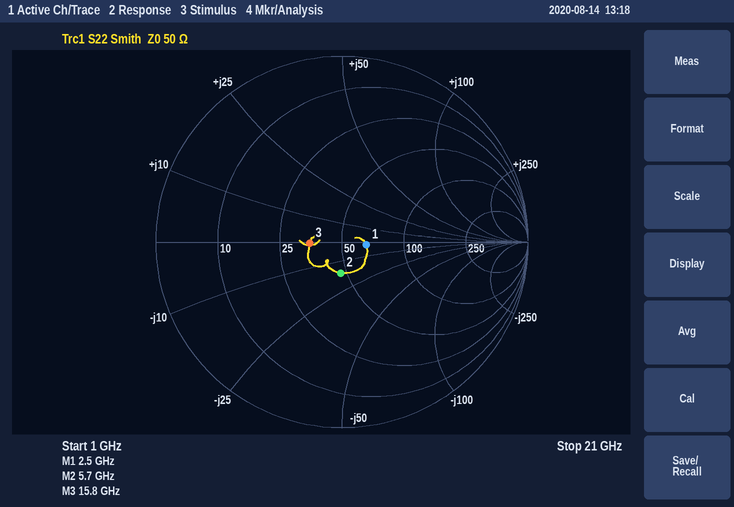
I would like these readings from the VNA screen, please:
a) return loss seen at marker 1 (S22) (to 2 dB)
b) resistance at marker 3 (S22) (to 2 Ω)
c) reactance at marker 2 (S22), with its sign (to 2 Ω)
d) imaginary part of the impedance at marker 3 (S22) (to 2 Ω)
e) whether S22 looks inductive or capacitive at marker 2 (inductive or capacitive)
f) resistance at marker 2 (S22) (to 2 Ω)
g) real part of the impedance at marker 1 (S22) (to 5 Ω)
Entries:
18 dB
36 Ω
-16 Ω
0 Ω
capacitive
46 Ω
65 Ω
